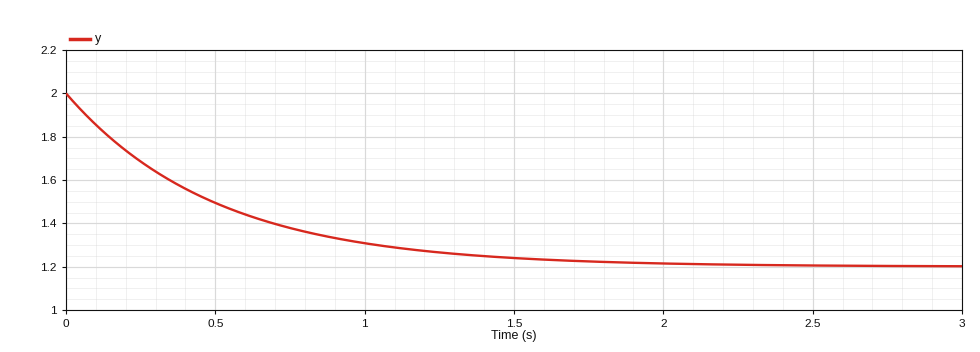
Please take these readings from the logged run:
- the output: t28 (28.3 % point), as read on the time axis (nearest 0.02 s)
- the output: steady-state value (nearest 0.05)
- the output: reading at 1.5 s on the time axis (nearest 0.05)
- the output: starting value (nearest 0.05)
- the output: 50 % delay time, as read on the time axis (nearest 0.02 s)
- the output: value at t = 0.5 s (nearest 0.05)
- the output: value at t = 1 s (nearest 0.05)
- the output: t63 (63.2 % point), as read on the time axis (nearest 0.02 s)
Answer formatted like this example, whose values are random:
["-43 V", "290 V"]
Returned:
["0.16 s", "1.20", "1.25", "2.00", "0.34 s", "1.50", "1.30", "0.50 s"]
